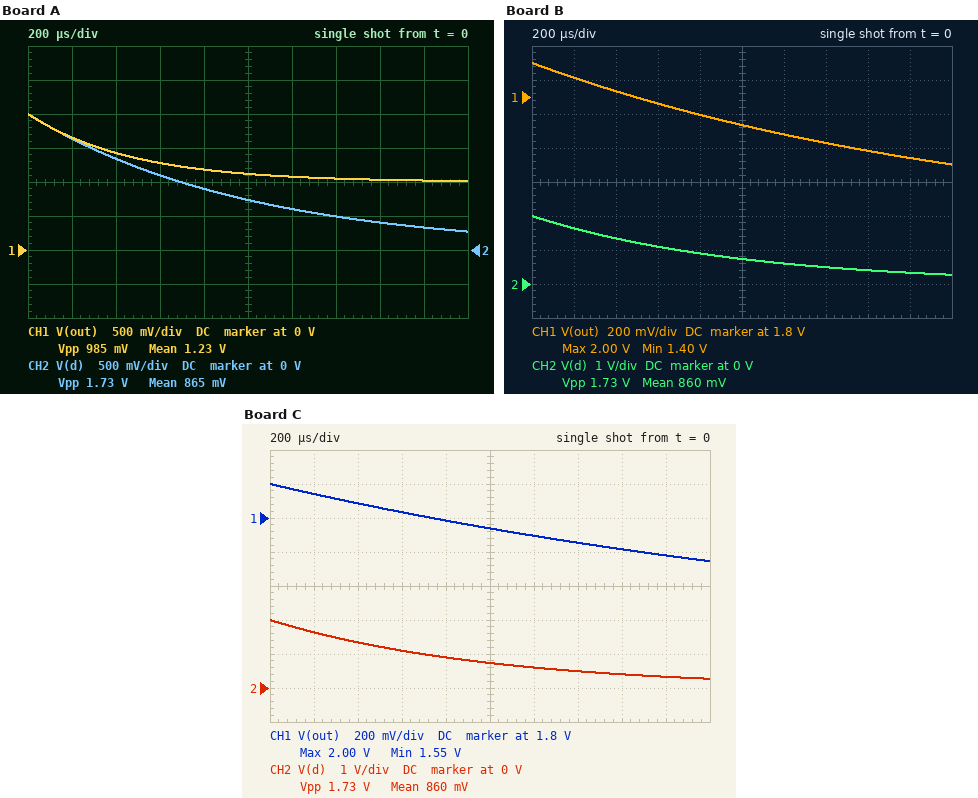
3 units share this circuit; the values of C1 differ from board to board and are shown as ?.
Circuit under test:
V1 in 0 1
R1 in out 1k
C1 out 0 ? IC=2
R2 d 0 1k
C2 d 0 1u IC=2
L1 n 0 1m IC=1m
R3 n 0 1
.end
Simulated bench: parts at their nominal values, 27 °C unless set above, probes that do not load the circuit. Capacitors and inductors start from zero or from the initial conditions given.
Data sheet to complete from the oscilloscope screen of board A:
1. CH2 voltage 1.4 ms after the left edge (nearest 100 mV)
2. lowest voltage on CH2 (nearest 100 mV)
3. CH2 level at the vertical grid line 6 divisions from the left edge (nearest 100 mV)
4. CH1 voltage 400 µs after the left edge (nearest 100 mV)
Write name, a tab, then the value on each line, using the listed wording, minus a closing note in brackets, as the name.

CH2 voltage 1.4 ms after the left edge	500 mV
lowest voltage on CH2	300 mV
CH2 level at the vertical grid line 6 divisions from the left edge	600 mV
CH1 voltage 400 µs after the left edge	1.4 V
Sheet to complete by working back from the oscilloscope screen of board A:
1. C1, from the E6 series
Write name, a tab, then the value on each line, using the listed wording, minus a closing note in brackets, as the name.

C1, from the E6 series	470 nF
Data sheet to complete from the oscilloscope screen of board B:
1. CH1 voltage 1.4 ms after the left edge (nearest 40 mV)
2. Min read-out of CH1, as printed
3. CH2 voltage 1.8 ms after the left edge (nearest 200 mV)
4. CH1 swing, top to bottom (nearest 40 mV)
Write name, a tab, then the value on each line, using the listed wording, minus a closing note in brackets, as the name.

CH1 voltage 1.4 ms after the left edge	1.52 V
Min read-out of CH1, as printed	1.40 V
CH2 voltage 1.8 ms after the left edge	400 mV
CH1 swing, top to bottom	600 mV
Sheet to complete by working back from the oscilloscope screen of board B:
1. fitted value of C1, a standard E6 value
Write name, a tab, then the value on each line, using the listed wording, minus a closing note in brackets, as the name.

fitted value of C1, a standard E6 value	2.2 µF
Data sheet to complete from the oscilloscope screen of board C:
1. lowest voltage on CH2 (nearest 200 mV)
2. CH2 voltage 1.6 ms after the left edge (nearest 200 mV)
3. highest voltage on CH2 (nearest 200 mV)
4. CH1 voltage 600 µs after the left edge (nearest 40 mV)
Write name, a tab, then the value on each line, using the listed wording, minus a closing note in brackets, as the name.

lowest voltage on CH2	200 mV
CH2 voltage 1.6 ms after the left edge	400 mV
highest voltage on CH2	2.0 V
CH1 voltage 600 µs after the left edge	1.84 V
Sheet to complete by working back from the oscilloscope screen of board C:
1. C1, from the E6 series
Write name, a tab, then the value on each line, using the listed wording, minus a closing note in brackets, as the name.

C1, from the E6 series	3.3 µF
